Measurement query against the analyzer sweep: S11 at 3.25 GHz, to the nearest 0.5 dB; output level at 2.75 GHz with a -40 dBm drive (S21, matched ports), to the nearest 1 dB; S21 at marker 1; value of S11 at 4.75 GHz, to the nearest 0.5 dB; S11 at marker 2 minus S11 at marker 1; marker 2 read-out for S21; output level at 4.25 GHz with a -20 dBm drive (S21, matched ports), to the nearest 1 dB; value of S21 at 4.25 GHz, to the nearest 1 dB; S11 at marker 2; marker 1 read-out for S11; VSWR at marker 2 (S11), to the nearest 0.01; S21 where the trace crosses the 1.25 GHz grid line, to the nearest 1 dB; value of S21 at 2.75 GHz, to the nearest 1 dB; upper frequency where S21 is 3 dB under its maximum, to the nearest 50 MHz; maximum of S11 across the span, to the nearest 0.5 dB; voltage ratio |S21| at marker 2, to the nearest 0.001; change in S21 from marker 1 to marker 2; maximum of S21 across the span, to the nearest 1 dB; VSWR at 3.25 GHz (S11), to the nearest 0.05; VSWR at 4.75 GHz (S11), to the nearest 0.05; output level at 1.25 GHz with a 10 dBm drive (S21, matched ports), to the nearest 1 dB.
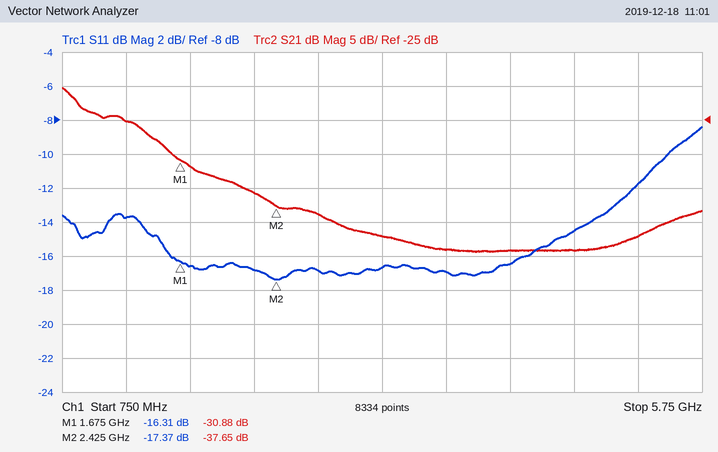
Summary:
-16.5 dB
-79 dBm
-30.88 dB
-14.5 dB
-1.06 dB
-37.65 dB
-64 dBm
-44 dB
-17.37 dB
-16.31 dB
1.31
-25 dB
-39 dB
900 MHz
-8.5 dB
0.013
-6.77 dB
-20 dB
1.35
1.45
-15 dBm
